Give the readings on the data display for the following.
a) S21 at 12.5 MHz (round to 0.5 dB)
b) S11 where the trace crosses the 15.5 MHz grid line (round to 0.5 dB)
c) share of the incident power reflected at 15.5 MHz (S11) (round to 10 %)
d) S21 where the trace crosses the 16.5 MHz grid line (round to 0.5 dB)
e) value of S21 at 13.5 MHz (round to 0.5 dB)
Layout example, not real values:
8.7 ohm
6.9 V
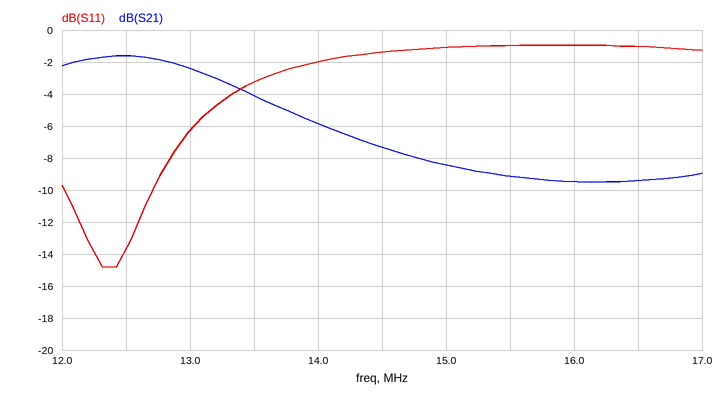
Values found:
-1.5 dB
-1.0 dB
80 %
-9.5 dB
-4.0 dB
